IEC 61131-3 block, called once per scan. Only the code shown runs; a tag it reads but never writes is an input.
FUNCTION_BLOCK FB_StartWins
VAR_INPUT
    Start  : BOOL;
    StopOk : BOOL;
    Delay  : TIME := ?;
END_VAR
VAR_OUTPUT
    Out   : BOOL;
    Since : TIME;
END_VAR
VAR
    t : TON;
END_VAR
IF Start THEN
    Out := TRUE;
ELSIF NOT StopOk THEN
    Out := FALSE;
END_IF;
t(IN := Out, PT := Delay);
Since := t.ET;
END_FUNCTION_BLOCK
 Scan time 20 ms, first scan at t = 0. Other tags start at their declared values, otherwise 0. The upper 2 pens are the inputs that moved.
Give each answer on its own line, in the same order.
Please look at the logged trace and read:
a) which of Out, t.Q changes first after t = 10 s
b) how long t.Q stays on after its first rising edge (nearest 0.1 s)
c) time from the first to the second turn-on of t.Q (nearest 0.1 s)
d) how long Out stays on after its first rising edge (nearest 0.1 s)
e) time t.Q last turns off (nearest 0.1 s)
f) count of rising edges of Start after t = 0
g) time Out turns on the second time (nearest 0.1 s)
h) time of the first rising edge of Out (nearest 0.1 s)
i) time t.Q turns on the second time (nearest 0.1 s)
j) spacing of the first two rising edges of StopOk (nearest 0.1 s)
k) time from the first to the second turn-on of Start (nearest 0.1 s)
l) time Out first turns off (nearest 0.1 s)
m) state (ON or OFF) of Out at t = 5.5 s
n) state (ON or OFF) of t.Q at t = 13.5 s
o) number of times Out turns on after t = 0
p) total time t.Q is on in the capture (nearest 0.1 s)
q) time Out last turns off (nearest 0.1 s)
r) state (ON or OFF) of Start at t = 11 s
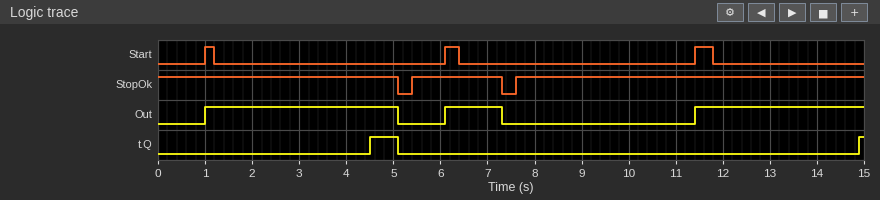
Out
0.6 s
10.4 s
4.1 s
5.1 s
3
6.1 s
1.0 s
14.9 s
2.2 s
5.1 s
5.1 s
OFF
OFF
3
0.7 s
7.3 s
OFF
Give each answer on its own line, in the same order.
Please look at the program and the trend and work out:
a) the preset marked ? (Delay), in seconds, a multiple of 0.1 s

3.5 s
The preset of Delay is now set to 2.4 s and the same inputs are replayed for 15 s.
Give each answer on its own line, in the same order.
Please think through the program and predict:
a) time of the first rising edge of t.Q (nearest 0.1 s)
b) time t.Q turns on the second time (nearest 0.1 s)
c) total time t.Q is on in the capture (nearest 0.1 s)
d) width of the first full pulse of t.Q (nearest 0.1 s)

3.4 s
13.8 s
2.9 s
1.7 s
